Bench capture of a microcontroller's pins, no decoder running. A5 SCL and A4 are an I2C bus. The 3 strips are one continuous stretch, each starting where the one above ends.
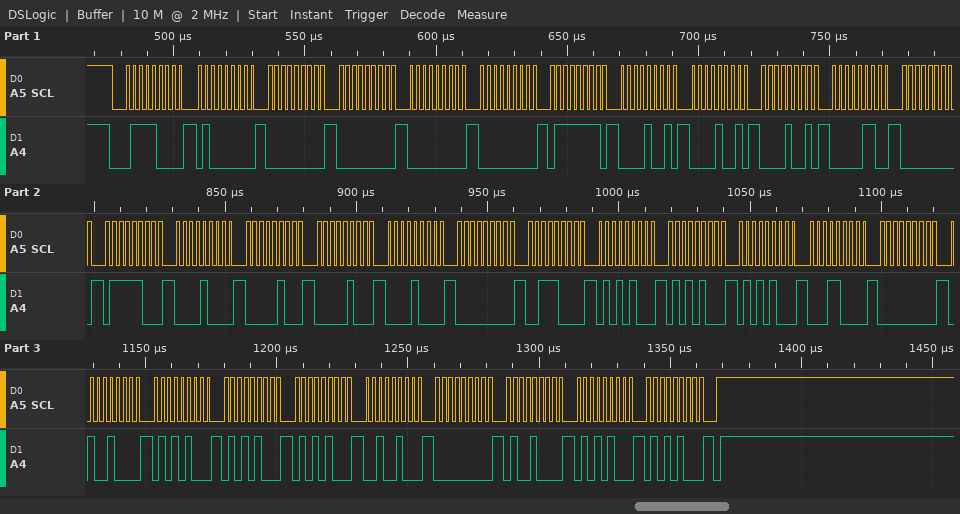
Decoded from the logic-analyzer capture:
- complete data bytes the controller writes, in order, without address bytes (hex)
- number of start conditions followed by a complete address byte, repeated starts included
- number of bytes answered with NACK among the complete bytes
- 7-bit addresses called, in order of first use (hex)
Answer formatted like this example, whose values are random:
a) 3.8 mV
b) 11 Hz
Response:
a) 40 00 00 00 00 7F 09 09 09 06 00 7C 08 04 04 08 00 38 54 54 54 18 00 48 54 54 54 24 00 48 54 54
b) 1
c) 0
d) 0x3C
